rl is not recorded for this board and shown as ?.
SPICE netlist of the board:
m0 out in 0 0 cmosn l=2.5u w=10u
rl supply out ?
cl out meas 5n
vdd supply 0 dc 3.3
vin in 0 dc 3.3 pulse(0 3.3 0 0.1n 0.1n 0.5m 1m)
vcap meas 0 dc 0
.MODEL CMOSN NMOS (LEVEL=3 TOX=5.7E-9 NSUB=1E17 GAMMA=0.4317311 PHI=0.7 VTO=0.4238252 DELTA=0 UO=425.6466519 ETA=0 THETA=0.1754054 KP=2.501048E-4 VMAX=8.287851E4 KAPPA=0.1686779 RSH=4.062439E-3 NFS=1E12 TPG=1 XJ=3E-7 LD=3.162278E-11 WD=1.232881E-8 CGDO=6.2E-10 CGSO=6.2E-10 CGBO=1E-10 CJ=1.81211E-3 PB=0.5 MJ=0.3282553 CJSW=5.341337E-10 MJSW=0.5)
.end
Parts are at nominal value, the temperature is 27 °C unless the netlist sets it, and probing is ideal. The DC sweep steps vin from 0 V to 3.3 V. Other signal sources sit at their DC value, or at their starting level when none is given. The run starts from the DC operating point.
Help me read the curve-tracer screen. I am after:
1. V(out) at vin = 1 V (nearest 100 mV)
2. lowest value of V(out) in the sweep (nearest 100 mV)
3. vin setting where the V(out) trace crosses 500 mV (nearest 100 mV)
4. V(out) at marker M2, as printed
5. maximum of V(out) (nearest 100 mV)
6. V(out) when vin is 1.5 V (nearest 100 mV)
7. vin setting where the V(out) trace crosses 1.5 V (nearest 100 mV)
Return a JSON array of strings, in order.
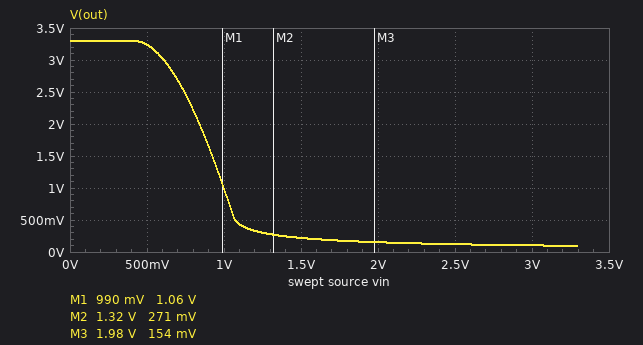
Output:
["1.0 V", "100 mV", "1.1 V", "271 mV", "3.3 V", "200 mV", "900 mV"]
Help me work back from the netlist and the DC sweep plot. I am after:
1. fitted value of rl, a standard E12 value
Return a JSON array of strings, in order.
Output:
["18 kΩ"]
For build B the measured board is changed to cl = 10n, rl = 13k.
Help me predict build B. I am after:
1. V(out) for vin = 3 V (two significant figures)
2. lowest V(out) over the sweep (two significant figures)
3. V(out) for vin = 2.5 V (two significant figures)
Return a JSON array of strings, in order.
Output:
["140 mV", "130 mV", "170 mV"]
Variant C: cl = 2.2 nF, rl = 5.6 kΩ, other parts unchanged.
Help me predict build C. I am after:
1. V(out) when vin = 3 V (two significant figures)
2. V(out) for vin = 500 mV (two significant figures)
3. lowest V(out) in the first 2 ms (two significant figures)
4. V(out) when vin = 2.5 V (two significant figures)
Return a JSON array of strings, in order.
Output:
["340 mV", "3.3 V", "310 mV", "400 mV"]
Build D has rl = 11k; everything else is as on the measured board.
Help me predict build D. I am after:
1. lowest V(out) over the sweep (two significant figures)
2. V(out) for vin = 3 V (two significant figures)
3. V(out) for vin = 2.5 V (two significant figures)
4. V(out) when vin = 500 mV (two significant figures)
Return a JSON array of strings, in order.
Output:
["160 mV", "170 mV", "200 mV", "3.3 V"]
